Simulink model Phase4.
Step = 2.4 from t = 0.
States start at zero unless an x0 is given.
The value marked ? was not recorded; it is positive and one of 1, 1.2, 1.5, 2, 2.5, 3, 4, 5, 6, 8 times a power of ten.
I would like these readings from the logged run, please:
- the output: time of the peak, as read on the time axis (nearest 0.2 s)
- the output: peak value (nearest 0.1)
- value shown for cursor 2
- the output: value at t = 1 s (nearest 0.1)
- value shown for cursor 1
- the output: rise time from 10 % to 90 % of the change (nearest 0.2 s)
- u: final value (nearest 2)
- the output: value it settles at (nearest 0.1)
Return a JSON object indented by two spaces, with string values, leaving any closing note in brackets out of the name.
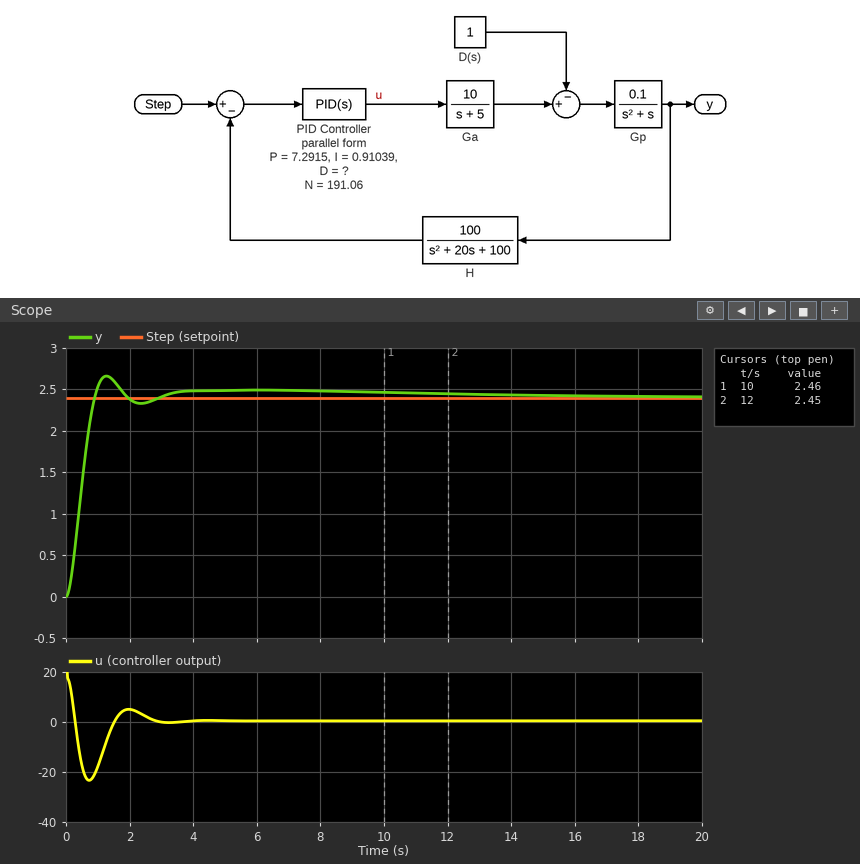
{
  "the output: time of the peak, as read on the time axis": "1.2 s",
  "the output: peak value": "2.7",
  "value shown for cursor 2": "2.45",
  "the output: value at t = 1 s": "2.5",
  "value shown for cursor 1": "2.46",
  "the output: rise time from 10 % to 90 % of the change": "0.6 s",
  "u: final value": "0",
  "the output: value it settles at": "2.4"
}
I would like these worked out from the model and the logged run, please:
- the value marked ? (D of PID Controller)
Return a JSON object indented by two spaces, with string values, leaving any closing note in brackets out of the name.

{
  "the value marked ?": "10"
}
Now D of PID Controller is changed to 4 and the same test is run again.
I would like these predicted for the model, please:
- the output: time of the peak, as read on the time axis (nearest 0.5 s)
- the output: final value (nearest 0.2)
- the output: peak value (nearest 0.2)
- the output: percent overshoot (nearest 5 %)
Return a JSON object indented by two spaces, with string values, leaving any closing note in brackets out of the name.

{
  "the output: time of the peak, as read on the time axis": "2.5 s",
  "the output: final value": "2.4",
  "the output: peak value": "3.0",
  "the output: percent overshoot": "25 %"
}
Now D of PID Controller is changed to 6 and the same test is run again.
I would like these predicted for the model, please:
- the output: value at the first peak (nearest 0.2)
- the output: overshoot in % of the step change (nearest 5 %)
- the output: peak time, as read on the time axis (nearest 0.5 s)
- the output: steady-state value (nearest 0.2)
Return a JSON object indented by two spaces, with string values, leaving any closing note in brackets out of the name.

{
  "the output: value at the first peak": "2.8",
  "the output: overshoot in % of the step change": "15 %",
  "the output: peak time, as read on the time axis": "2.0 s",
  "the output: steady-state value": "2.4"
}
